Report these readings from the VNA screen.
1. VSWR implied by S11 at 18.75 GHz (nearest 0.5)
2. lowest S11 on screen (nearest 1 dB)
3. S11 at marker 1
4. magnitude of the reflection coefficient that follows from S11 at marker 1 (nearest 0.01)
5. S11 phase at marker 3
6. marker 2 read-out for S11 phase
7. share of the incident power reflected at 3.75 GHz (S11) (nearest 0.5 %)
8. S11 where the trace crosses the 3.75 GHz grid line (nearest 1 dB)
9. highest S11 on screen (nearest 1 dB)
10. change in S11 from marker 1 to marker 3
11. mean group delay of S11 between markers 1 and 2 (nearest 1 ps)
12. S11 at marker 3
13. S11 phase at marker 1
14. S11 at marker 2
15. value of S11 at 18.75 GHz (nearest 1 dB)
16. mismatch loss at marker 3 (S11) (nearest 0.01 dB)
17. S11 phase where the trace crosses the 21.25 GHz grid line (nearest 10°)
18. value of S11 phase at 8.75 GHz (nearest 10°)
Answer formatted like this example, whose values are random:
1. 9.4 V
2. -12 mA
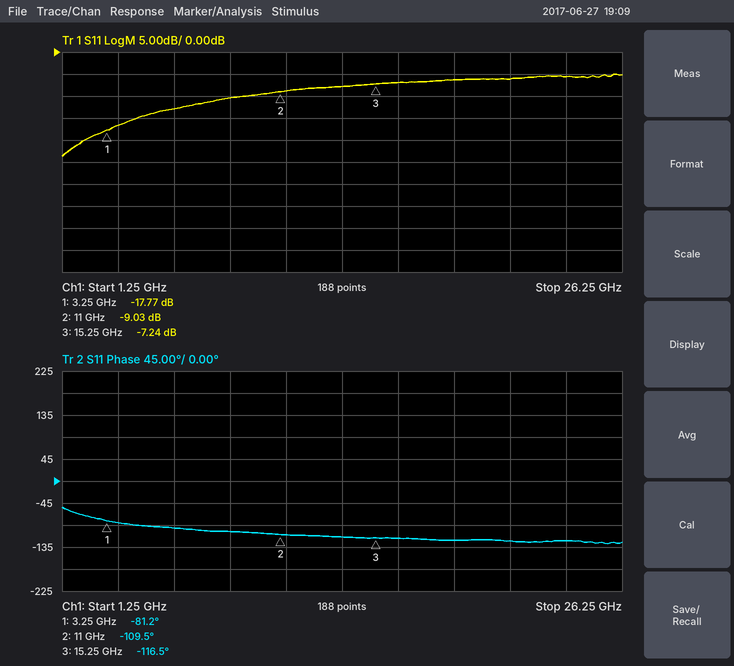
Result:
1. 3.0
2. -24 dB
3. -17.77 dB
4. 0.13
5. -116.5°
6. -109.5°
7. 2.0 %
8. -17 dB
9. -5 dB
10. 10.53 dB
11. 10 ps
12. -7.24 dB
13. -81.2°
14. -9.03 dB
15. -6 dB
16. 0.91 dB
17. -120°
18. -100°
